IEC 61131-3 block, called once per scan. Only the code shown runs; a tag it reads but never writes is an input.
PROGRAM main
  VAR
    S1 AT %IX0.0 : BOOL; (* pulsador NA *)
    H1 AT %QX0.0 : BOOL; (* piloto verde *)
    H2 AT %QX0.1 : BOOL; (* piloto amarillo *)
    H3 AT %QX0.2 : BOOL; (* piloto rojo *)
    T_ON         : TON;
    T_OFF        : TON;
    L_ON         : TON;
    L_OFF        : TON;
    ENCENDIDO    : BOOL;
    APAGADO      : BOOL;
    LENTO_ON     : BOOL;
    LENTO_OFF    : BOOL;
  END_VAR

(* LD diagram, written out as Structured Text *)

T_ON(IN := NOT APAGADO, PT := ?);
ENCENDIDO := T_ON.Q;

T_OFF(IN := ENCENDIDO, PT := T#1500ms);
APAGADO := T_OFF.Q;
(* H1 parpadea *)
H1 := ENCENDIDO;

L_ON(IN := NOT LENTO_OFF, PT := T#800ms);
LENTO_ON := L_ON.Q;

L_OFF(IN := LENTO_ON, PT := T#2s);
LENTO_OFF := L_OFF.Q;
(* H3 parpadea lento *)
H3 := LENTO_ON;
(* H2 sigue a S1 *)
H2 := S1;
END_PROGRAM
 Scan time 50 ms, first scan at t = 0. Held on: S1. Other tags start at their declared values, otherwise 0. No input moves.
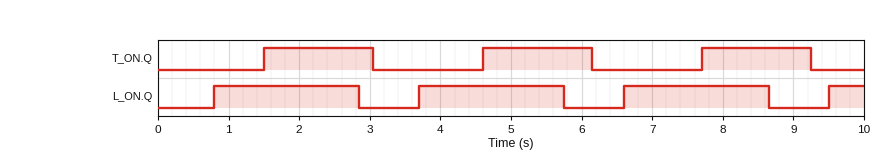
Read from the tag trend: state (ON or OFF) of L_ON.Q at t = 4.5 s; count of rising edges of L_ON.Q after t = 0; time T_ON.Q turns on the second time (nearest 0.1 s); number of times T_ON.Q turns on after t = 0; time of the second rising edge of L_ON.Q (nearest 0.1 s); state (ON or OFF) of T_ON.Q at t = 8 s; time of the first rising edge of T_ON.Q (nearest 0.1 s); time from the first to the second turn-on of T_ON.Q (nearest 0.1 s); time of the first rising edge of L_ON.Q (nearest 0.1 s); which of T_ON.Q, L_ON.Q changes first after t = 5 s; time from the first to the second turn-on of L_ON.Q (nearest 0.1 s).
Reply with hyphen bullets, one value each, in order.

- ON
- 4
- 4.6 s
- 3
- 3.7 s
- ON
- 1.5 s
- 3.1 s
- 0.8 s
- L_ON.Q
- 2.9 s
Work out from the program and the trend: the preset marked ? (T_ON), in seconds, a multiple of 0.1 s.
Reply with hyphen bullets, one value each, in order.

- 1.5 s
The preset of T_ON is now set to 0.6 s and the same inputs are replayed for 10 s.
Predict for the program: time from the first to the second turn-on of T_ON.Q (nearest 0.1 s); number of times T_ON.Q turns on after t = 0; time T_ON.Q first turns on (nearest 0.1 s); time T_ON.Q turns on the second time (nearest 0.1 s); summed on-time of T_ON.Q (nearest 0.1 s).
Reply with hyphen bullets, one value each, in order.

- 2.2 s
- 5
- 0.6 s
- 2.8 s
- 6.8 s
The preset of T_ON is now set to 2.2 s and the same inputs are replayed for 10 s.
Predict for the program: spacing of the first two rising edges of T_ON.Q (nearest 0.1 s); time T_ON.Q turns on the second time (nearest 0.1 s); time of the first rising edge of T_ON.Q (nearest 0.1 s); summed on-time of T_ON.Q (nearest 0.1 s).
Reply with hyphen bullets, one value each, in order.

- 3.8 s
- 6.0 s
- 2.2 s
- 3.3 s
